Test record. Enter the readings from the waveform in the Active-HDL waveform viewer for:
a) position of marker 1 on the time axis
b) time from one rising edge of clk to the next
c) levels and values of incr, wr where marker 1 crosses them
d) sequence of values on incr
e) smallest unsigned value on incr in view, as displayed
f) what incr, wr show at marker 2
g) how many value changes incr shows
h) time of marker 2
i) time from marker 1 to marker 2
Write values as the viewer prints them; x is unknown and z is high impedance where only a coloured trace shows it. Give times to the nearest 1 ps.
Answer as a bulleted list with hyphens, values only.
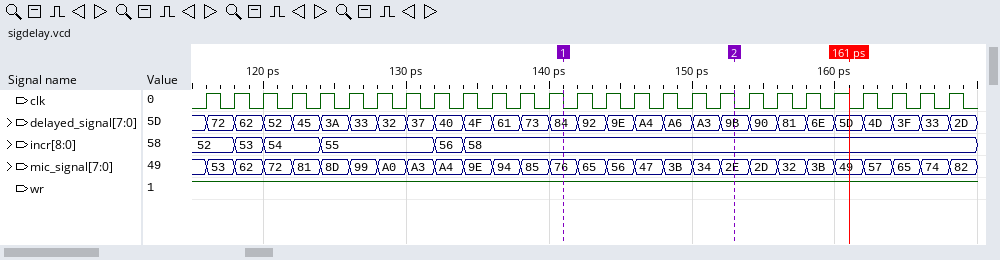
- 141 ps
- 2 ps
- incr=58, wr=1
- 52, 53, 54, 55, 56, 58
- 52
- incr=58, wr=1
- 5
- 153 ps
- 12 ps
